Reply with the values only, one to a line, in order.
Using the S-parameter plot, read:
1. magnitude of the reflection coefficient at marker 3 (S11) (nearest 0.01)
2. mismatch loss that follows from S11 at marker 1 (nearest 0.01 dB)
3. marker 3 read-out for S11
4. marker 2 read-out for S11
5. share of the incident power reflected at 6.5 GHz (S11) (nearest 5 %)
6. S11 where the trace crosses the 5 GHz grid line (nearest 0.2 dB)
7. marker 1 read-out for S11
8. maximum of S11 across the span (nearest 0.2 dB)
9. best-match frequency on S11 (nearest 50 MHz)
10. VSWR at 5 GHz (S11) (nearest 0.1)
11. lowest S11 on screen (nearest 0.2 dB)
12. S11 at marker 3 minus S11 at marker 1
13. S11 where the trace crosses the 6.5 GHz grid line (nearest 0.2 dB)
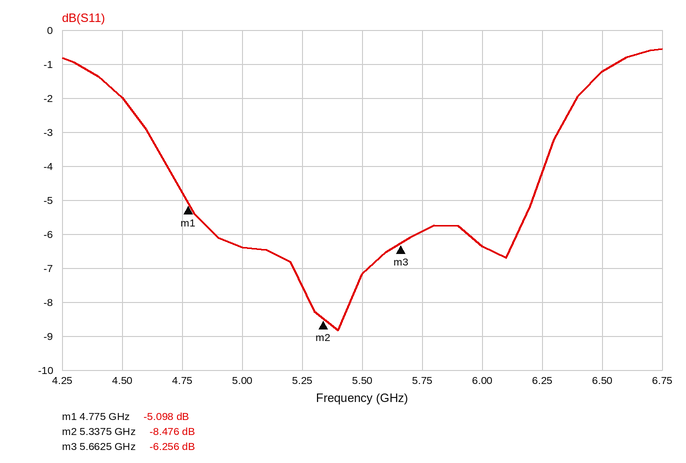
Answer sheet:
0.49
1.61 dB
-6.256 dB
-8.476 dB
75 %
-6.4 dB
-5.098 dB
-0.6 dB
5.40 GHz
2.8
-8.8 dB
-1.158 dB
-1.2 dB
